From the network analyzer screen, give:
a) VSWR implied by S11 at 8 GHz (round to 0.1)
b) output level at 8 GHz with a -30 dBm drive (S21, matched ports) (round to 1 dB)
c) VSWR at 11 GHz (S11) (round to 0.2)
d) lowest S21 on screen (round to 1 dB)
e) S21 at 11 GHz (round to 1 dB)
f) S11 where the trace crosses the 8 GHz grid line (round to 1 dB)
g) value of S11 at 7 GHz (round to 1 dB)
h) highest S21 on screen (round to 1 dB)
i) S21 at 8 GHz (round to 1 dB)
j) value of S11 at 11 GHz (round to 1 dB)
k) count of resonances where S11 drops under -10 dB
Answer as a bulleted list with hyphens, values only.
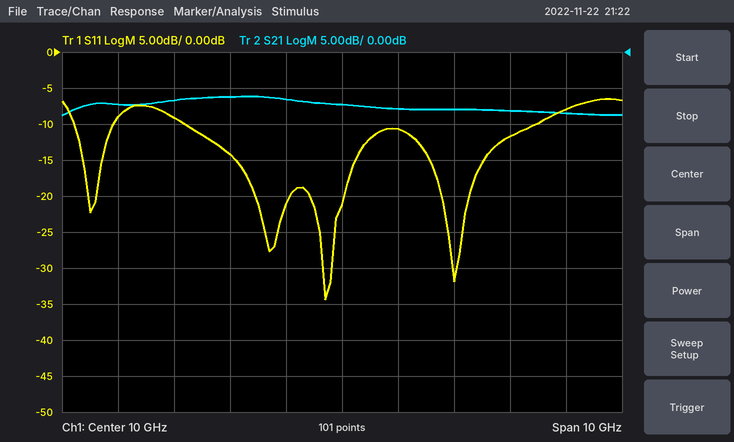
- 1.5
- -36 dBm
- 1.8
- -9 dB
- -8 dB
- -14 dB
- -9 dB
- -6 dB
- -6 dB
- -11 dB
- 4
